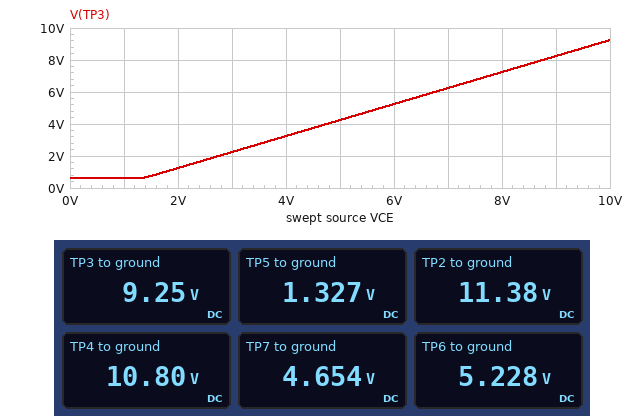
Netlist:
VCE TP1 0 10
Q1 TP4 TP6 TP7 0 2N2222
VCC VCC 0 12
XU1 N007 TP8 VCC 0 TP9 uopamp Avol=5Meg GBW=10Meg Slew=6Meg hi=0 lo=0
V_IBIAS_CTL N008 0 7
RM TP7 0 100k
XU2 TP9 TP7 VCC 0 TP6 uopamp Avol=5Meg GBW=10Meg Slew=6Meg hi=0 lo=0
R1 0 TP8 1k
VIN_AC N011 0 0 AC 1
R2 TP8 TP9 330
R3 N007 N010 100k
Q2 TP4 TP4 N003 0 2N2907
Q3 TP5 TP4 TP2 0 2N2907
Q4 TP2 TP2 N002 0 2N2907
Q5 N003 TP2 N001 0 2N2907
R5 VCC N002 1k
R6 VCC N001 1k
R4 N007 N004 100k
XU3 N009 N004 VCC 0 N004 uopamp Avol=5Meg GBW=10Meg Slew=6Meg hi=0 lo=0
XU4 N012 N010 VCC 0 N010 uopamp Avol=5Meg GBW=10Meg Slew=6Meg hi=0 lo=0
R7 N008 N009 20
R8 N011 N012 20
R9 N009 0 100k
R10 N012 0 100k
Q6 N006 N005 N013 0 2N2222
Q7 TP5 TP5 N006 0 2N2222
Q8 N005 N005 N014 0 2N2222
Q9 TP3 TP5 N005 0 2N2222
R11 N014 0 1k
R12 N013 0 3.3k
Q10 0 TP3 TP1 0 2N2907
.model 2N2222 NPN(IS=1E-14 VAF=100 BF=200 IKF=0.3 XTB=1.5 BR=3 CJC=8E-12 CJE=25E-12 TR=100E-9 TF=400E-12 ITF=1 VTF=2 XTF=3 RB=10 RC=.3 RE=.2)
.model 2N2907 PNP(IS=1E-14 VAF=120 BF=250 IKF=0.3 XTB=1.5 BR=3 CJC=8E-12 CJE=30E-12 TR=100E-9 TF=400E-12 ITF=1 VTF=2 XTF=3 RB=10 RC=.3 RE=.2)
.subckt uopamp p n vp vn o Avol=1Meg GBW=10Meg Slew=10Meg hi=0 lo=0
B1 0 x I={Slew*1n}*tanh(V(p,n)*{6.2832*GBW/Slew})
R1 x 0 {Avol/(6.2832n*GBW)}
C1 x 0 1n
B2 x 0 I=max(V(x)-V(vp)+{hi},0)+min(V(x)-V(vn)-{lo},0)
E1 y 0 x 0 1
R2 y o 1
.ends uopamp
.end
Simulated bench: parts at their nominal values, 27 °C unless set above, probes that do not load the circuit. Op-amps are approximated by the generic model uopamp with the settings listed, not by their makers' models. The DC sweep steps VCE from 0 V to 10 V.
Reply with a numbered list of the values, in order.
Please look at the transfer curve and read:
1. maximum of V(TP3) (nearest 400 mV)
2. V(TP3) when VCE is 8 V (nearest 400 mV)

1. 9.2 V
2. 7.2 V
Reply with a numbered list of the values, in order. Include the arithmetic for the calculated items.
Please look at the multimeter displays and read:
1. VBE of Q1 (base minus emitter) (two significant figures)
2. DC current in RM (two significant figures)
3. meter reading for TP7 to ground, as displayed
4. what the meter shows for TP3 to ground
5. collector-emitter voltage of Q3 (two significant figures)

1. 5.228 V - 4.654 V = 570 mV
2. (4.654 V) / 100 kΩ = 47 µA
3. 4.654 V
4. 9.25 V
5. 1.327 V - 11.38 V = -10 V
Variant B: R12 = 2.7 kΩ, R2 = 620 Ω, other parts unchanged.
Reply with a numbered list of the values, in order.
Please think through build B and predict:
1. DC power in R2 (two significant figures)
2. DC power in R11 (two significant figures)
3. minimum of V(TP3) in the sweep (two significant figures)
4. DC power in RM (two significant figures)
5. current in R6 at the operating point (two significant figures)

1. 7.6 mW
2. 17 µW
3. 610 mV
4. 320 µW
5. 56 µA
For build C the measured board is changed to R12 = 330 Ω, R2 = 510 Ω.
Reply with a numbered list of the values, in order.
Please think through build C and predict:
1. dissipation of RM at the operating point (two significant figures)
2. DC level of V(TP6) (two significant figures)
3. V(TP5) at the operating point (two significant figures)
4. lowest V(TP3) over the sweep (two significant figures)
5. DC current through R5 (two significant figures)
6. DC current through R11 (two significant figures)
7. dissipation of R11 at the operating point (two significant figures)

1. 280 µW
2. 5.9 V
3. 1.2 V
4. 580 mV
5. 53 µA
6. 31 µA
7. 970 nW
